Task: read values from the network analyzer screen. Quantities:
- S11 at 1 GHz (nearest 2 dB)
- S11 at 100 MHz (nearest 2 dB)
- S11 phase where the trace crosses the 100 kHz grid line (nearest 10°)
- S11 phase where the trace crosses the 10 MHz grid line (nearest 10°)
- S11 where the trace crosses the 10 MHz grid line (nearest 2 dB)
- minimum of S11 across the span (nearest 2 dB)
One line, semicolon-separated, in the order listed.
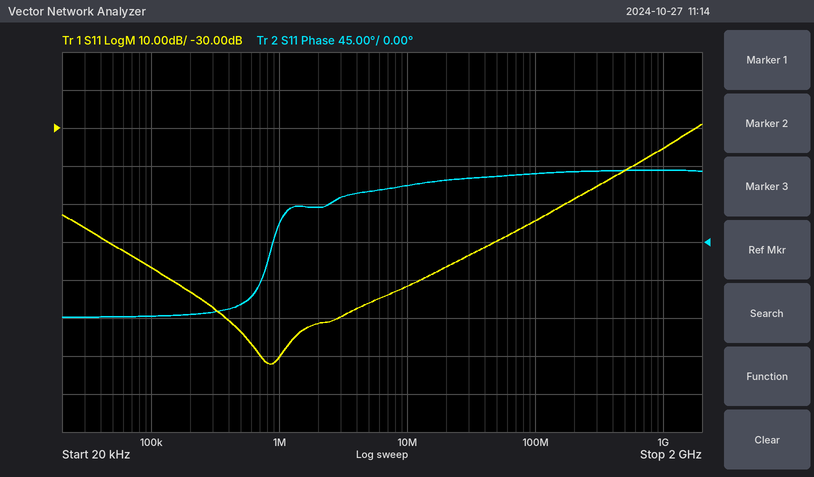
-36 dB; -54 dB; -90°; 70°; -72 dB; -92 dB
